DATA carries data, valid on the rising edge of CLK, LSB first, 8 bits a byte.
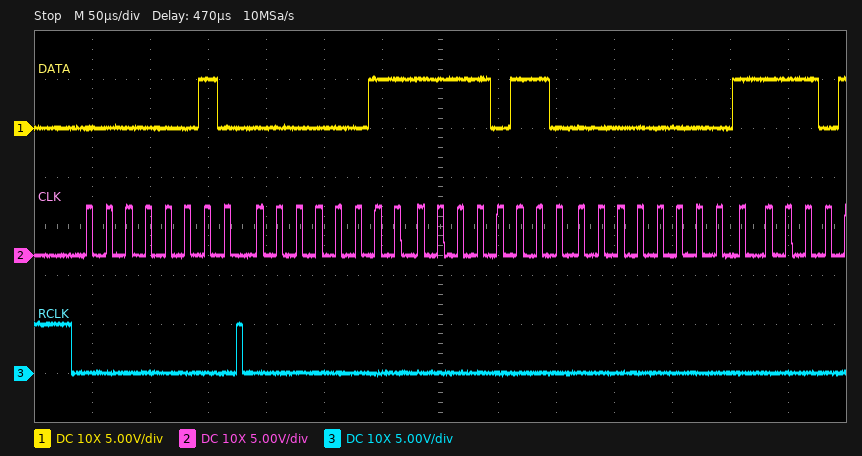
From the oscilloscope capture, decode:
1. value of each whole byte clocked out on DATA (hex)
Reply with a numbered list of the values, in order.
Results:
1. 40 C0 6F 00
